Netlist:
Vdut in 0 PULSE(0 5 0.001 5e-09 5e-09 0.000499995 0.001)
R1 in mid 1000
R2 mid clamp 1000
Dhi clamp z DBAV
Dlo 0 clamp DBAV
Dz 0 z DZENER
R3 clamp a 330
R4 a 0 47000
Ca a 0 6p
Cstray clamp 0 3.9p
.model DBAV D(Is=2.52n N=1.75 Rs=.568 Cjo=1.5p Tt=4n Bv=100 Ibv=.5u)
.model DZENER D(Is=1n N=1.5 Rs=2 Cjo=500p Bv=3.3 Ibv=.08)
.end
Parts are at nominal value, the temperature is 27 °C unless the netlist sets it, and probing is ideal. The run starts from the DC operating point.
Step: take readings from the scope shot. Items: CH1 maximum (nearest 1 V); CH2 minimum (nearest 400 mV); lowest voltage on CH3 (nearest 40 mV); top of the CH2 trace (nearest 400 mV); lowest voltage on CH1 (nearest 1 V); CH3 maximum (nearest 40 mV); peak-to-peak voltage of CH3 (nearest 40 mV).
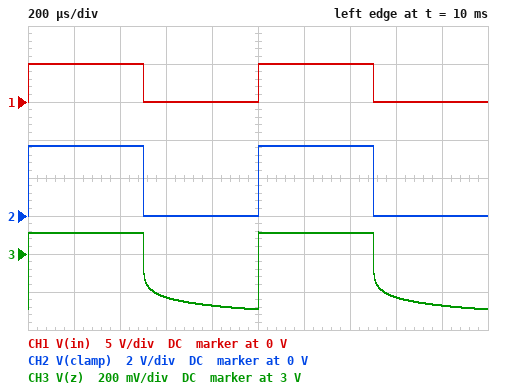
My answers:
5 V
0 V
2.72 V
3.6 V
0 V
3.12 V
400 mV
